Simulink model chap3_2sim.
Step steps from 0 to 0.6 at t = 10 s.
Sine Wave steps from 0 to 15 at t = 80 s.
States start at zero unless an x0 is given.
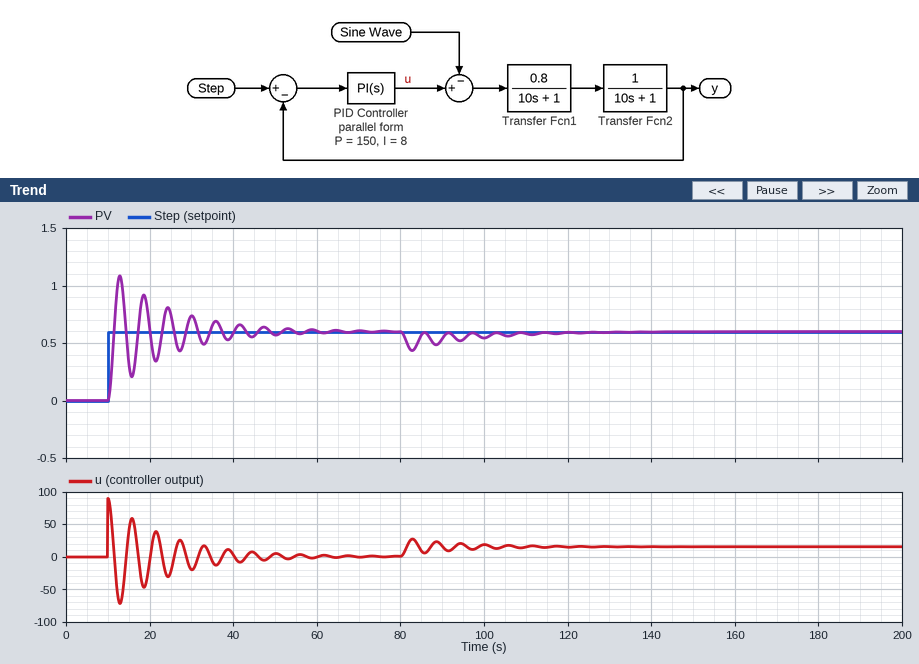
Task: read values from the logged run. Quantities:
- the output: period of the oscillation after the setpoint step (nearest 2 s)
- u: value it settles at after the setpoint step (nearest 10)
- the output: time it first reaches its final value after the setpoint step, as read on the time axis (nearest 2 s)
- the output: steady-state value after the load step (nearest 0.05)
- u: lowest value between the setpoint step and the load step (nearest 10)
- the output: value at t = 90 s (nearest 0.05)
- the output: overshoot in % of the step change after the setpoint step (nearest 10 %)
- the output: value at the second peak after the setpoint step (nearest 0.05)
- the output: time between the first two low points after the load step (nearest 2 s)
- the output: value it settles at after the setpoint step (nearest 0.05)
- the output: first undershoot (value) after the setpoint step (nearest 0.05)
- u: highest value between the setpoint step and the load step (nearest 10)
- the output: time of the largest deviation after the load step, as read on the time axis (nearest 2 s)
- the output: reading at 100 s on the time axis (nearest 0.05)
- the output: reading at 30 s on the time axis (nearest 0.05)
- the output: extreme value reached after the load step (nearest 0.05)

6 s
0
12 s
0.60
-70
0.55
80 %
0.90
6 s
0.60
0.20
90
82 s
0.55
0.75
0.45
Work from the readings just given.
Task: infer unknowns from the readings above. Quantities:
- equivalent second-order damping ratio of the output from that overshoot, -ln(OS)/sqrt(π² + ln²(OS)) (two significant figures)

0.071
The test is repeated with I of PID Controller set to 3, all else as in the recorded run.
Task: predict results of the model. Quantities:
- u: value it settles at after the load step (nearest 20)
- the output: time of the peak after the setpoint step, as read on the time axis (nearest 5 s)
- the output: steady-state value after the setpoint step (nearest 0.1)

20
15 s
0.6
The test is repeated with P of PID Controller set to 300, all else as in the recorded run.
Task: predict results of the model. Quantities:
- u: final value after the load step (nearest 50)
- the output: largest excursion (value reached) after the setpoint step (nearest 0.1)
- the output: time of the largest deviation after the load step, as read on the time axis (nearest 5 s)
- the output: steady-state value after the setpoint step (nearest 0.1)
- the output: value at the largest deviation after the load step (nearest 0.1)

0
1.1
80 s
0.6
0.5
